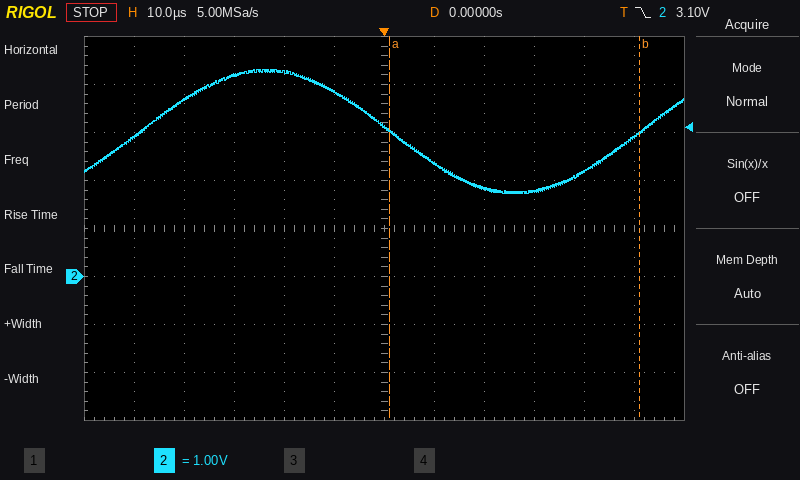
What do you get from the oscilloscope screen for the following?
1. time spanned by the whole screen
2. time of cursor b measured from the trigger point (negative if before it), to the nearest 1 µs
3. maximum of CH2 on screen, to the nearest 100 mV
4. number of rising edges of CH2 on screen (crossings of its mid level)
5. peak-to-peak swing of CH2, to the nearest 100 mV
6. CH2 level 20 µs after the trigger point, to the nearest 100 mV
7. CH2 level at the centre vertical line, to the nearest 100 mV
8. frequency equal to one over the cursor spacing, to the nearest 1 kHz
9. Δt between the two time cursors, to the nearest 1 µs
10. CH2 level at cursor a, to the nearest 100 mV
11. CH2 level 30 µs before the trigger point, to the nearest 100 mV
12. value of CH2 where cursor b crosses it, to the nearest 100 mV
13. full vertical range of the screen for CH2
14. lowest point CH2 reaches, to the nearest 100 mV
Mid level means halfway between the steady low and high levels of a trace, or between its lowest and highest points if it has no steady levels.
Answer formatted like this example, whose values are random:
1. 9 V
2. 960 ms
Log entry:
1. 120 µs
2. +51 µs
3. 4.3 V
4. 2
5. 2.6 V
6. 1.8 V
7. 3.1 V
8. 20 kHz
9. 50 µs
10. 3.0 V
11. 4.2 V
12. 3.0 V
13. 8 V
14. 1.7 V
